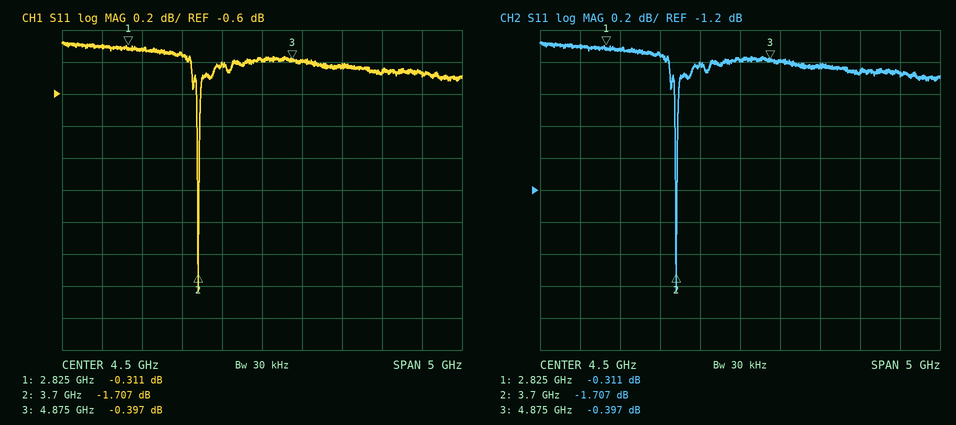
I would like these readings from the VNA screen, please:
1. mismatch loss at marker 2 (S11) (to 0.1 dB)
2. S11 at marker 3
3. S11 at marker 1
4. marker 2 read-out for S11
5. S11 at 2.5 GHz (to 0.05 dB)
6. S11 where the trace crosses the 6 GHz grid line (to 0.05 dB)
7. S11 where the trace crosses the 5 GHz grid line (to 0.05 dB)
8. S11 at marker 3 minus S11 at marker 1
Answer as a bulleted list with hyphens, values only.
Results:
- 4.9 dB
- -0.397 dB
- -0.311 dB
- -1.707 dB
- -0.30 dB
- -0.45 dB
- -0.40 dB
- -0.086 dB
